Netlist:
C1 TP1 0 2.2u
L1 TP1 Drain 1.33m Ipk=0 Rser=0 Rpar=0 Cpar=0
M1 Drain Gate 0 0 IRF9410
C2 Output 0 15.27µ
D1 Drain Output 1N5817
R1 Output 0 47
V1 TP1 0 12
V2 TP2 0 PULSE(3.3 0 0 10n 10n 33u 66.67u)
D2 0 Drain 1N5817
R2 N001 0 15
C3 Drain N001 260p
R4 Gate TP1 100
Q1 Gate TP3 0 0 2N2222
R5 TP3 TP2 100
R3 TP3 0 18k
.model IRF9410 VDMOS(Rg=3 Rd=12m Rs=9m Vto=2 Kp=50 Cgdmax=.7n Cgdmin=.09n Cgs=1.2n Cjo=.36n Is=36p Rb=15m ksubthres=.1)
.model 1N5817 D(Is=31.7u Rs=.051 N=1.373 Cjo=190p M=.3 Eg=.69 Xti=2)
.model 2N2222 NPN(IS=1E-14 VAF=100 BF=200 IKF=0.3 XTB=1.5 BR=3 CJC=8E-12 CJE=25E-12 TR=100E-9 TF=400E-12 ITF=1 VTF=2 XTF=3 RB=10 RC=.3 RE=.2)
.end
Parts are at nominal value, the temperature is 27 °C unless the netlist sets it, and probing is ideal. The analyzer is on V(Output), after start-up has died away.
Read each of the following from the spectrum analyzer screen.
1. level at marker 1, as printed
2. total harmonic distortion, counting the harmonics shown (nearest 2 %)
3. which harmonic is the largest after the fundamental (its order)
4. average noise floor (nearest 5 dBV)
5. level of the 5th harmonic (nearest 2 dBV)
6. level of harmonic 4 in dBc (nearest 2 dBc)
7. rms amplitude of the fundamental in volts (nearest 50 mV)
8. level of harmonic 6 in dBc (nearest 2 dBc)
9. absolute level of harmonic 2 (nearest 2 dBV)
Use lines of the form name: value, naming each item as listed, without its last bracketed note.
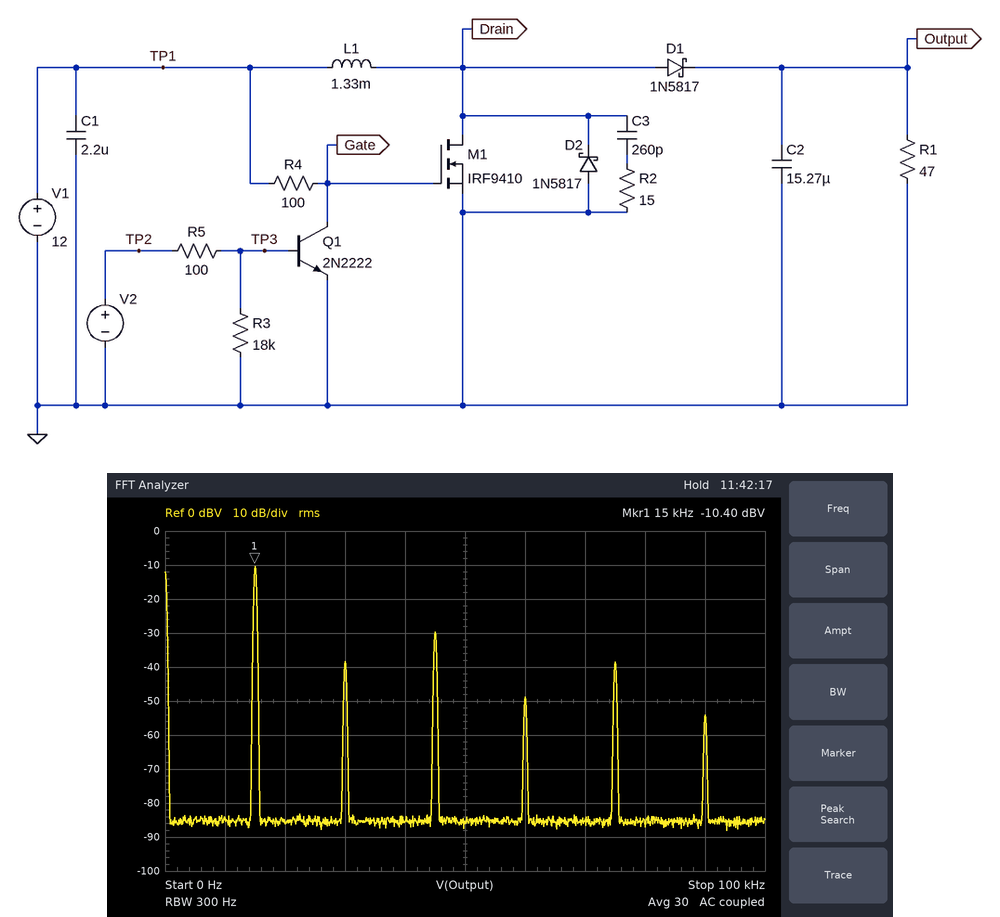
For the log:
level at marker 1, as printed: -10.40 dBV
total harmonic distortion, counting the harmonics shown: 12 %
which harmonic is the largest after the fundamental: 3
average noise floor: -85 dBV
level of the 5th harmonic: -38 dBV
level of harmonic 4 in dBc: -38 dBc
rms amplitude of the fundamental in volts: 300 mV
level of harmonic 6 in dBc: -44 dBc
absolute level of harmonic 2: -38 dBV
